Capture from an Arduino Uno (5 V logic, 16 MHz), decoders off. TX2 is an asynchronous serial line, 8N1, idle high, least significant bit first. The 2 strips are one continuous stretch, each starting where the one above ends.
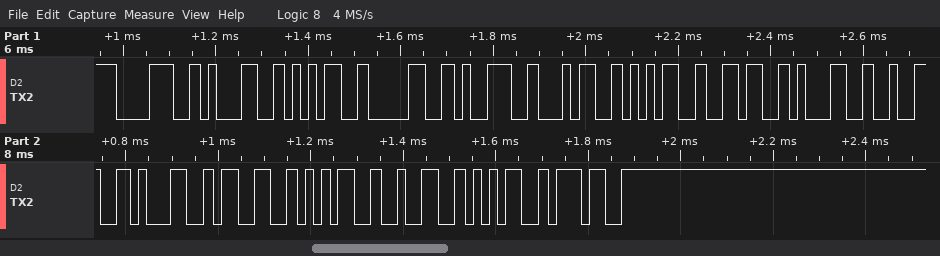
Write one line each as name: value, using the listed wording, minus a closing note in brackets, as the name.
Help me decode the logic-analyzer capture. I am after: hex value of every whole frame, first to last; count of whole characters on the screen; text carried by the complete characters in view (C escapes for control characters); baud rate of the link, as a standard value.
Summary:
hex value of every whole frame, first to last: 38 31 35 30 39 34 35 36 31 32 31 33 35 32 35 37
count of whole characters on the screen: 16
text carried by the complete characters in view: "8150945612135257"
baud rate of the link, as a standard value: 57600 baud
